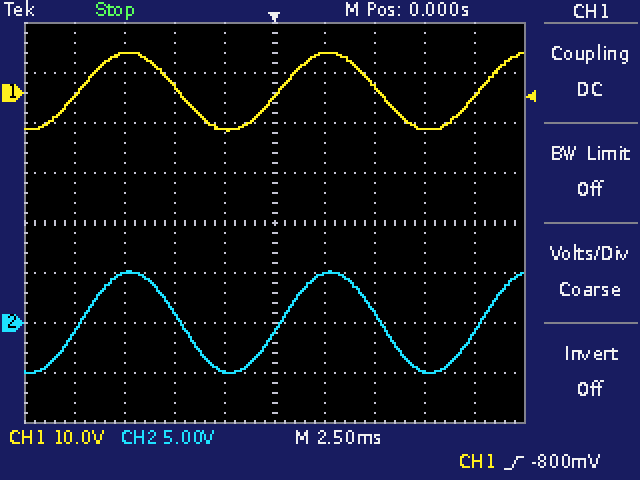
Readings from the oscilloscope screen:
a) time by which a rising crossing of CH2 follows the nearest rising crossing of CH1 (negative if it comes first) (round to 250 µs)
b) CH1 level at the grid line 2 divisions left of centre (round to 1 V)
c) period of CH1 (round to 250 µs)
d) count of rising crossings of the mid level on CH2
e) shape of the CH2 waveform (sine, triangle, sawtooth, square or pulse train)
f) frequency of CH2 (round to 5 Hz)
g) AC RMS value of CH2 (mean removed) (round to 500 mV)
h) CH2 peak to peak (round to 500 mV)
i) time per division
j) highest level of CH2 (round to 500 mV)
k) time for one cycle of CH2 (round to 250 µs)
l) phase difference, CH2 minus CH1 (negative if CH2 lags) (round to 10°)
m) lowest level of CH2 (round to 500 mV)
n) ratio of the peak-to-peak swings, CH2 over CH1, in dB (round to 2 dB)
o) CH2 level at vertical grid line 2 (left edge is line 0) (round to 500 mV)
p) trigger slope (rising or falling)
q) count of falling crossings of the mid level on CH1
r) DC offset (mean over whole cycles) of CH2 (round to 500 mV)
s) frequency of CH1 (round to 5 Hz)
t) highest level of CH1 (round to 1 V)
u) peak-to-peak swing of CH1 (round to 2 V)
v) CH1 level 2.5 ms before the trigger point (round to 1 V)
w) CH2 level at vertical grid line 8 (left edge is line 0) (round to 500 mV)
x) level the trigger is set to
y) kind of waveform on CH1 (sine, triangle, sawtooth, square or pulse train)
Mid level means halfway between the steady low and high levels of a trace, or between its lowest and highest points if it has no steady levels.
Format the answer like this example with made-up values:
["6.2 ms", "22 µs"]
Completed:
["0.00 ms", "1 V", "10.00 ms", "3", "sine", "100 Hz", "3.5 V", "10.0 V", "2.5 ms", "5.0 V", "10.00 ms", "0°", "-5.0 V", "-4 dB", "5.0 V", "rising", "2", "0.0 V", "100 Hz", "8 V", "16 V", "-7 V", "-5.0 V", "-800 mV", "sine"]
